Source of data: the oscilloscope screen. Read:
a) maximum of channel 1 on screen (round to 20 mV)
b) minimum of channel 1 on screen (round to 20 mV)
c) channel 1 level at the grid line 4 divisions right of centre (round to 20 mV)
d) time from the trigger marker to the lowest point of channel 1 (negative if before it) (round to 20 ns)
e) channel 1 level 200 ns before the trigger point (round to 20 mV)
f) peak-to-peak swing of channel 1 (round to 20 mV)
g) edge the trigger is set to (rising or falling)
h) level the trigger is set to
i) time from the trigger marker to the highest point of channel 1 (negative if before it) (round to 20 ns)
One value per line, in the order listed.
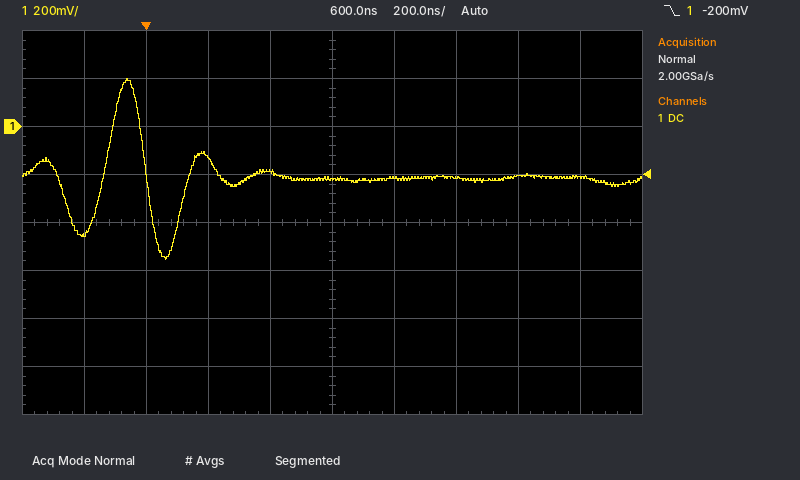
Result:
200 mV
-560 mV
-220 mV
+60 ns
-440 mV
760 mV
falling
-200 mV
-60 ns
